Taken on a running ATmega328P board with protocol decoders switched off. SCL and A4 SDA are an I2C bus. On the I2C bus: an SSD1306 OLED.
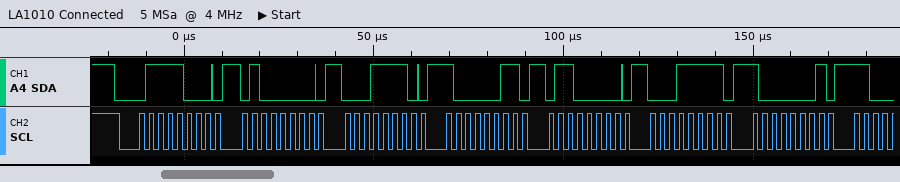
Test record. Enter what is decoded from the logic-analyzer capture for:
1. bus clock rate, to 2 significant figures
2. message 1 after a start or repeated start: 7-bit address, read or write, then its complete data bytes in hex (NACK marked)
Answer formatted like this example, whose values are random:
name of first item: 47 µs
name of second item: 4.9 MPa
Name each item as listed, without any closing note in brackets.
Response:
bus clock rate, to 2 significant figures: 400 kHz
message 1 after a start or repeated start: 7-bit address, read or write, then its complete data bytes in hex: 0x3C write: 40 1E 83 60 1F 81
